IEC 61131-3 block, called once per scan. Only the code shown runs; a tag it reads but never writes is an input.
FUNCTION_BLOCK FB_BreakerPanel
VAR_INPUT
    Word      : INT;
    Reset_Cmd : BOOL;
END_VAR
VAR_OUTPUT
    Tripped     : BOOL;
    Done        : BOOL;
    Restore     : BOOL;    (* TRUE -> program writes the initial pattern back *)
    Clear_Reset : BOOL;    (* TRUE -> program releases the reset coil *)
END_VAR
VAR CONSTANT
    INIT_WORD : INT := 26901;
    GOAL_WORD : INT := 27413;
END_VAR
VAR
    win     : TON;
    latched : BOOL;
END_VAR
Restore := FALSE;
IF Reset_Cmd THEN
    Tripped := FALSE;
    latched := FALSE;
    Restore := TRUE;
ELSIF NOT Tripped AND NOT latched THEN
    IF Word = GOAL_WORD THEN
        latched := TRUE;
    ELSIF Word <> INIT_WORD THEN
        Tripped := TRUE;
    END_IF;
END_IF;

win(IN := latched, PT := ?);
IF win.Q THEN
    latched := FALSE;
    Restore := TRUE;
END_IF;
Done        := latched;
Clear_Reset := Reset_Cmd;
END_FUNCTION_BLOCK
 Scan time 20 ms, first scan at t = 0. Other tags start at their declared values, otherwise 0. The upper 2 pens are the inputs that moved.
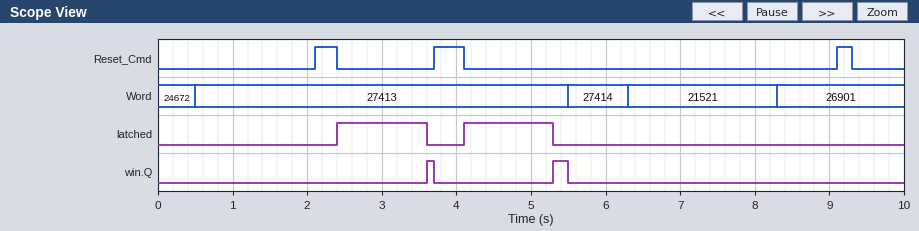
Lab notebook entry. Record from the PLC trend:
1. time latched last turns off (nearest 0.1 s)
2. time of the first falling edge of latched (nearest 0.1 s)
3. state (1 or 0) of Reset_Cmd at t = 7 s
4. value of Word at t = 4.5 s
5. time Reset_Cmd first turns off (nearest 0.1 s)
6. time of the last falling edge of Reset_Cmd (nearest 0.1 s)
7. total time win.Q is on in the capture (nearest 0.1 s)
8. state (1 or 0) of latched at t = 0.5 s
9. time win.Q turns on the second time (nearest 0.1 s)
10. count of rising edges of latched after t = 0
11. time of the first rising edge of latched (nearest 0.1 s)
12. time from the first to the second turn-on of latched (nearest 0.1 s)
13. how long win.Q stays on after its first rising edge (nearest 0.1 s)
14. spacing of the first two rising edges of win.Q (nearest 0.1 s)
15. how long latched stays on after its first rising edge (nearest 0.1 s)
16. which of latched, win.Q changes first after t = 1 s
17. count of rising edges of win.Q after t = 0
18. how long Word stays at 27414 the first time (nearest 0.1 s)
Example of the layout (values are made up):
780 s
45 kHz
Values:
5.3 s
3.6 s
0
27413
2.4 s
9.3 s
0.3 s
0
5.3 s
2
2.4 s
1.7 s
0.1 s
1.7 s
1.2 s
latched
2
0.8 s
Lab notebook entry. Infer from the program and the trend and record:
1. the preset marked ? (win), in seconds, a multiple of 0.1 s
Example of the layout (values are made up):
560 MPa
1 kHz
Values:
1.2 s
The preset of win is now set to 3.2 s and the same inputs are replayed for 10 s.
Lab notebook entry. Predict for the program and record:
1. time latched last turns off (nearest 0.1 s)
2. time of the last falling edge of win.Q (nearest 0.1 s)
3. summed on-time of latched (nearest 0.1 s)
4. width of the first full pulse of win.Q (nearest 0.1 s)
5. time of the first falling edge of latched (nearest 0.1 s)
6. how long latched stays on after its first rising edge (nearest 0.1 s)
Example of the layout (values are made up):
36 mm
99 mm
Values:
7.3 s
7.3 s
4.5 s
0.0 s
3.7 s
1.3 s
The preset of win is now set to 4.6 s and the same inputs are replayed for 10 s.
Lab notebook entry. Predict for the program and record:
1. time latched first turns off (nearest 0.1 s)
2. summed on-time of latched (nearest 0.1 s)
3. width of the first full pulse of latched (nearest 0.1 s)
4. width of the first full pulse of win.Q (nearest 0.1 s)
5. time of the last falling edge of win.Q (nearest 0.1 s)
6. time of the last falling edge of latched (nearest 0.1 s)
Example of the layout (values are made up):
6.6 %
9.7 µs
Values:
3.7 s
5.9 s
1.3 s
0.0 s
8.7 s
8.7 s
